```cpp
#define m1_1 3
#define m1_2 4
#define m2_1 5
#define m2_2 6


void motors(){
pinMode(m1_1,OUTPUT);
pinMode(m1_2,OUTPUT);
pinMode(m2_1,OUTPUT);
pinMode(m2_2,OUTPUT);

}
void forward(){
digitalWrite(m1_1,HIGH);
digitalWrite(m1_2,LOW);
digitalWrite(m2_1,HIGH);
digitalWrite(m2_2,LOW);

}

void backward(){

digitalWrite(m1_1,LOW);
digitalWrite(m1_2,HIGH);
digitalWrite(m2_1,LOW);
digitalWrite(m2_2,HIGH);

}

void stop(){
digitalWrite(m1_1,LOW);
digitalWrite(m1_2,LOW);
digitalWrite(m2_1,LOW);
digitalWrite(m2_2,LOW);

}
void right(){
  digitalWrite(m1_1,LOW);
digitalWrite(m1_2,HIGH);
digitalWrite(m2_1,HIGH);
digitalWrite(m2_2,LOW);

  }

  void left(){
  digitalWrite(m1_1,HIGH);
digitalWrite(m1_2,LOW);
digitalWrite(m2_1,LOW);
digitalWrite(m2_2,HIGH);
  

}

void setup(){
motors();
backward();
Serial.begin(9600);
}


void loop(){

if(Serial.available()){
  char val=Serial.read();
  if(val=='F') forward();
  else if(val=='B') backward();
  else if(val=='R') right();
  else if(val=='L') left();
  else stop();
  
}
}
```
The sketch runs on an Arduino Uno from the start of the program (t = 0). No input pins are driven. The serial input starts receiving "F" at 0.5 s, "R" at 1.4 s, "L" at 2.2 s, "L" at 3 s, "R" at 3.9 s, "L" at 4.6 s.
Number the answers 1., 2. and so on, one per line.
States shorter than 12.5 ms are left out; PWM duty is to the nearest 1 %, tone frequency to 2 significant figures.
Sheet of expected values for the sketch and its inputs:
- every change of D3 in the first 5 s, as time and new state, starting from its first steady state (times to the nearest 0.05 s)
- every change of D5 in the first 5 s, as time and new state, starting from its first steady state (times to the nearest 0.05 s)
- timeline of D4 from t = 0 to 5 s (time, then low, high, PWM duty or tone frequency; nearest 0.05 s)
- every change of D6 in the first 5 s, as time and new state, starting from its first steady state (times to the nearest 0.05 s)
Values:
1. 0 s low; 0.5 s high; 1.4 s low; 2.2 s high; 3.9 s low; 4.6 s high
2. 0 s low; 0.5 s high; 2.2 s low; 3.9 s high; 4.6 s low
3. 0 s high; 0.5 s low; 1.4 s high; 2.2 s low; 3.9 s high; 4.6 s low
4. 0 s high; 0.5 s low; 2.2 s high; 3.9 s low; 4.6 s high
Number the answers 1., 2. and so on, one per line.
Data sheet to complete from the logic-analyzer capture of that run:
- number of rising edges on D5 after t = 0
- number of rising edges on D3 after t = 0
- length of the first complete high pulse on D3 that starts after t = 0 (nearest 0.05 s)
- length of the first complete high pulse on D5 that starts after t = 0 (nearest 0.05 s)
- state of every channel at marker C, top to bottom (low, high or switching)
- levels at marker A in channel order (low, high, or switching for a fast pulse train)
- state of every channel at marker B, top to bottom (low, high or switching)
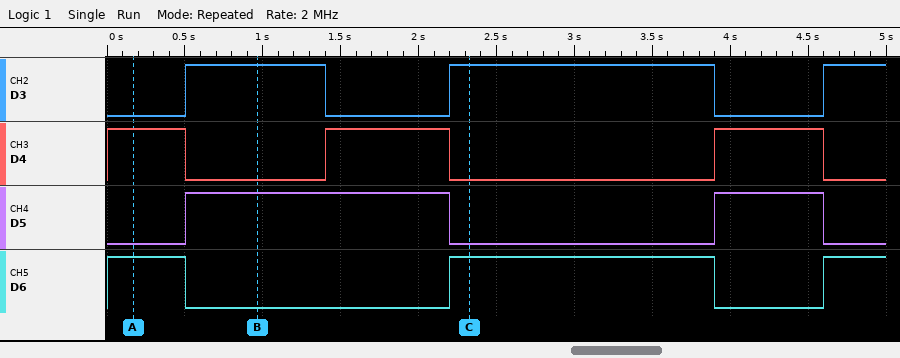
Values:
1. 2
2. 3
3. 0.90 s
4. 1.70 s
5. D3 high, D4 low, D5 low, D6 high
6. D3 low, D4 high, D5 low, D6 high
7. D3 high, D4 low, D5 high, D6 low
